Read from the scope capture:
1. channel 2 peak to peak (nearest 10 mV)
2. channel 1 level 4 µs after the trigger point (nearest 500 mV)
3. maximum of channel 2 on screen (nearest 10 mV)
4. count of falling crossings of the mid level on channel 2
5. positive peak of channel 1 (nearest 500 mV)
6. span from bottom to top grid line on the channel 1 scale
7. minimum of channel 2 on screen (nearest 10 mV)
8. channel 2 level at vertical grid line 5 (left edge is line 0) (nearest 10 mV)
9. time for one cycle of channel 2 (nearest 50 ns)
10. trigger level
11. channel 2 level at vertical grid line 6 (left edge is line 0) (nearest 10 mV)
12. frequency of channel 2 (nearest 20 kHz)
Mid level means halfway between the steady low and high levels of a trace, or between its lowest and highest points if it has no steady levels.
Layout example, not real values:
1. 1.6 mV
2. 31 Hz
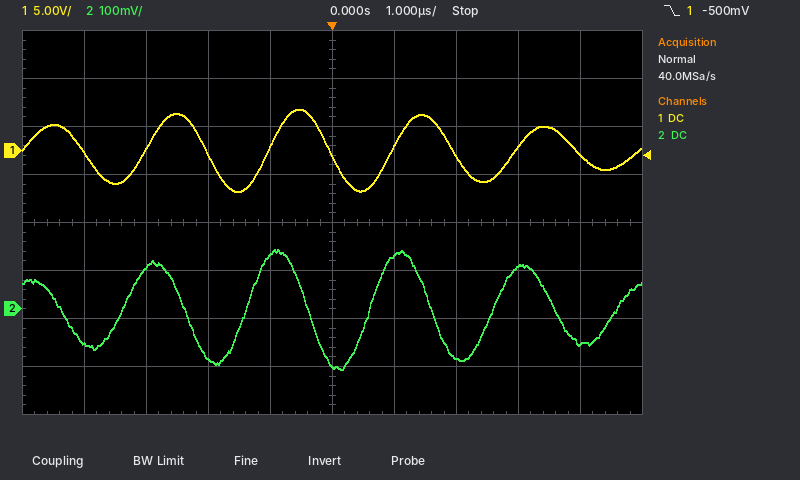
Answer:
1. 250 mV
2. -500 mV
3. 120 mV
4. 5
5. 4.5 V
6. 40 V
7. -130 mV
8. -120 mV
9. 2.00 µs
10. -500 mV
11. 110 mV
12. 500 kHz
